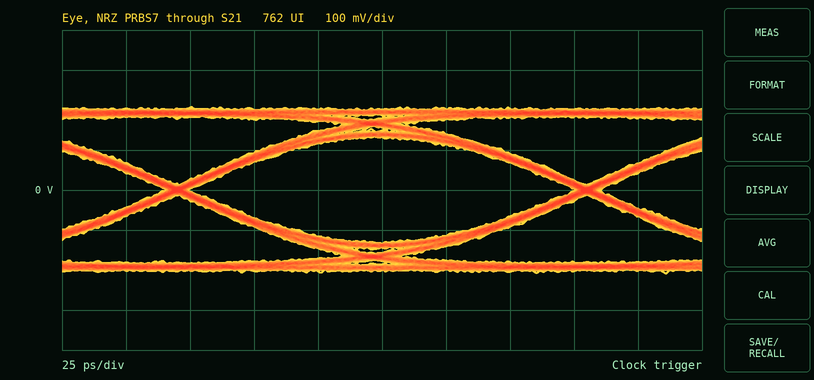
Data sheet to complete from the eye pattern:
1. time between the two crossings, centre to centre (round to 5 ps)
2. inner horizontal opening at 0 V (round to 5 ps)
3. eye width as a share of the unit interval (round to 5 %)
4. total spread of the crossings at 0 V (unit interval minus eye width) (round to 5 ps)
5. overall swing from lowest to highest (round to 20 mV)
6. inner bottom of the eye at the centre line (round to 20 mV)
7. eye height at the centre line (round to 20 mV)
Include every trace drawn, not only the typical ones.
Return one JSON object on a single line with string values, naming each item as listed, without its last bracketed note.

{"time between the two crossings, centre to centre": "160 ps", "inner horizontal opening at 0 V": "150 ps", "eye width as a share of the unit interval": "95 %", "total spread of the crossings at 0 V (unit interval minus eye width)": "10 ps", "overall swing from lowest to highest": "420 mV", "inner bottom of the eye at the centre line": "-140 mV", "eye height at the centre line": "260 mV"}
